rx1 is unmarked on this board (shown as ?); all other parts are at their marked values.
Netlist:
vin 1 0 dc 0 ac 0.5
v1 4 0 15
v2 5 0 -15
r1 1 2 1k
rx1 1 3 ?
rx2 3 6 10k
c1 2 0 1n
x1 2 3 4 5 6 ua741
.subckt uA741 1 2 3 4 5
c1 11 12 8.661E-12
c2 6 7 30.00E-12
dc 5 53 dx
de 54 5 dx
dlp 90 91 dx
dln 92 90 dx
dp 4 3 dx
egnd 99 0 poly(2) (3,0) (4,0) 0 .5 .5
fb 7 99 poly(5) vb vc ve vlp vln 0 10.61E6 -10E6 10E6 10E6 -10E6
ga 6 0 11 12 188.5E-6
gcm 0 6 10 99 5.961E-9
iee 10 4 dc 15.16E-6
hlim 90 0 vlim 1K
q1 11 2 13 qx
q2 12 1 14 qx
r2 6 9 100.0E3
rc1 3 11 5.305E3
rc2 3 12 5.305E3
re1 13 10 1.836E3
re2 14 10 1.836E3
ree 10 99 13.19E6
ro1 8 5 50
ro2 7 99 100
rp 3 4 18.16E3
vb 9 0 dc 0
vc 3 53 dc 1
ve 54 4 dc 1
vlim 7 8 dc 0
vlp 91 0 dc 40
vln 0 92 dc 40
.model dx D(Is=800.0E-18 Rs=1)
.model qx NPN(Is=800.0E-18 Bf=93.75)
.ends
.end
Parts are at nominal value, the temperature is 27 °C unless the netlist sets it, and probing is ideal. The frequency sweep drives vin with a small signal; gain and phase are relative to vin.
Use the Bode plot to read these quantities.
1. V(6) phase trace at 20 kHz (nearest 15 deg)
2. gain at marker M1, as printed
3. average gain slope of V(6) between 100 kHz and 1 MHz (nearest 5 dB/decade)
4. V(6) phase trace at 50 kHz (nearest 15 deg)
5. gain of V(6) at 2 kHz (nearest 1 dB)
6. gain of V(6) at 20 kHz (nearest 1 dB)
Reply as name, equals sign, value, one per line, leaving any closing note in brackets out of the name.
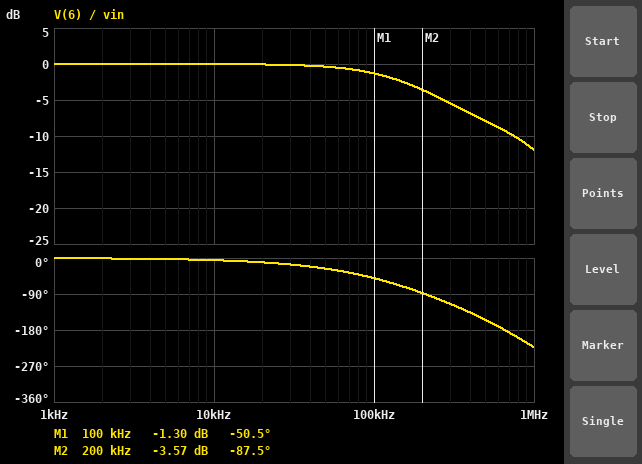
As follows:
V(6) phase trace at 20 kHz = -15 deg
gain at marker M1, as printed = -1.30 dB
average gain slope of V(6) between 100 kHz and 1 MHz = -10 dB/decade
V(6) phase trace at 50 kHz = -30 deg
gain of V(6) at 2 kHz = 0 dB
gain of V(6) at 20 kHz = 0 dB
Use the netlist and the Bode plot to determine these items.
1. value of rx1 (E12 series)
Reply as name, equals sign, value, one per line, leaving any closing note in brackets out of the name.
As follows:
value of rx1 = 33 kΩ
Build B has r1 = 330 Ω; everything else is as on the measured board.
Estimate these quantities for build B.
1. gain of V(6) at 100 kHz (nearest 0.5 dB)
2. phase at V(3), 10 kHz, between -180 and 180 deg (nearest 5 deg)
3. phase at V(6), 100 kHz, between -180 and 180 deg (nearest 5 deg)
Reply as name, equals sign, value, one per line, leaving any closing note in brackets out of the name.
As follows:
gain of V(6) at 100 kHz = 0 dB
phase at V(3), 10 kHz, between -180 and 180 deg = 0 deg
phase at V(6), 100 kHz, between -180 and 180 deg = -25 deg
